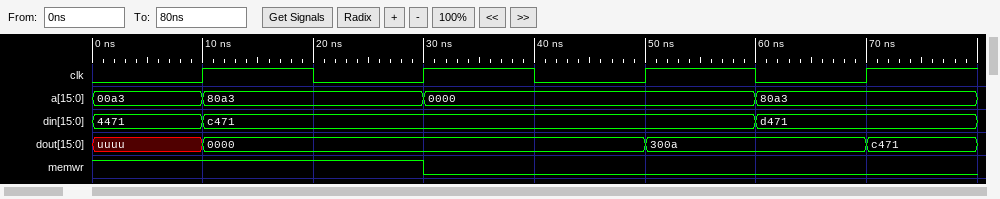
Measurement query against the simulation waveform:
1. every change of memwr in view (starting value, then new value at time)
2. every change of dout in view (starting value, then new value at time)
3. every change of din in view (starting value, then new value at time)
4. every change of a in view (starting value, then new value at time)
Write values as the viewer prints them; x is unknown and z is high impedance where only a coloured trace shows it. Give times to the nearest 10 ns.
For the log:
1, 0 at 30 ns
uuuu, 0000 at 10 ns, 300a at 50 ns, c471 at 70 ns
4471, c471 at 10 ns, d471 at 60 ns
00a3, 80a3 at 10 ns, 0000 at 30 ns, 80a3 at 60 ns
